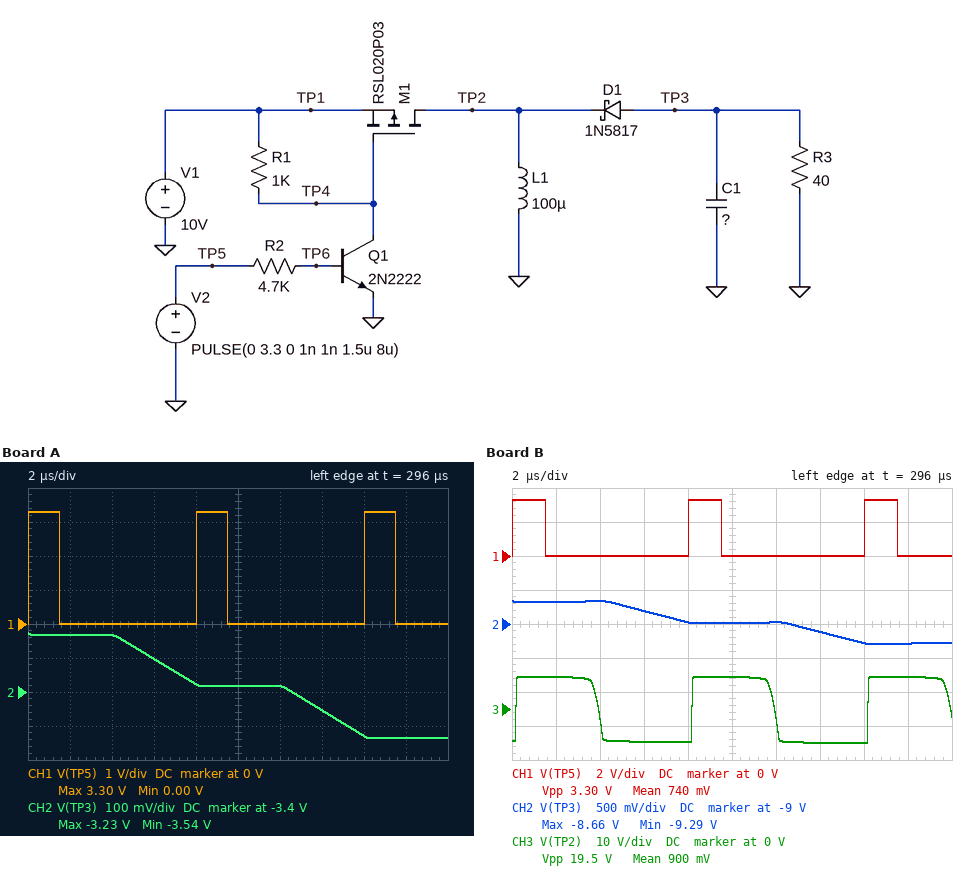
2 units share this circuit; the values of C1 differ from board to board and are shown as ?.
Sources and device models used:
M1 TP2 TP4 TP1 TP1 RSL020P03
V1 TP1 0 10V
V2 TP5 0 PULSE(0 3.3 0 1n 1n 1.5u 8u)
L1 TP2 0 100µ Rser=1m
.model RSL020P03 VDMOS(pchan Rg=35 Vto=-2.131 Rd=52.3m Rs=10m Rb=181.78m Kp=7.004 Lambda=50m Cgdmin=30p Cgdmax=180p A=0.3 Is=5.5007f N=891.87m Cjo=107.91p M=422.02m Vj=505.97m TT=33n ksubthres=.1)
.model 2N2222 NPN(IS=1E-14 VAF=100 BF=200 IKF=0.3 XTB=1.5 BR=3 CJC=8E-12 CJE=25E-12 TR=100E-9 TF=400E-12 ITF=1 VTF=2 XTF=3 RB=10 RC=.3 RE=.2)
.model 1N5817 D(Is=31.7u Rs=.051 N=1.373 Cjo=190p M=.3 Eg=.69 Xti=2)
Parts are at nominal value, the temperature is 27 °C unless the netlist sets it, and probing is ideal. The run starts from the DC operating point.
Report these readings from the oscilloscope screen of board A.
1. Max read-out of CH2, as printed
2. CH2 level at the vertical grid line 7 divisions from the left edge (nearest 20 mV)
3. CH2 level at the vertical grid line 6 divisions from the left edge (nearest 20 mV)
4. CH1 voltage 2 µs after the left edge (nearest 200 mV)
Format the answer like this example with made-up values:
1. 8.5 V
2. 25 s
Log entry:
1. -3.23 V
2. -3.46 V
3. -3.38 V
4. 0 V
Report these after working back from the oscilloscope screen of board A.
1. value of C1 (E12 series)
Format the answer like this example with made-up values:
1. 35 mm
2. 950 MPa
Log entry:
1. 270 µF
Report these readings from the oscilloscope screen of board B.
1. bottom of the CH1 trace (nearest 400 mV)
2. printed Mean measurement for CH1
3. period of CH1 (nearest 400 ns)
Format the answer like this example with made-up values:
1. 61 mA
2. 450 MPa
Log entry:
1. 0 V
2. 740 mV
3. 8.0 µs
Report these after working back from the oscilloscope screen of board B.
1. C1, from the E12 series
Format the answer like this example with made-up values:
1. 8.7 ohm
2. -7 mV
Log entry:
1. 82 µF
